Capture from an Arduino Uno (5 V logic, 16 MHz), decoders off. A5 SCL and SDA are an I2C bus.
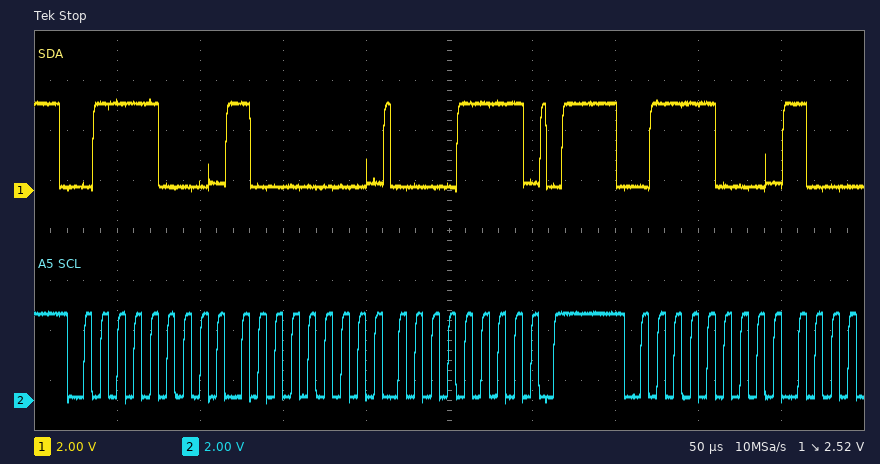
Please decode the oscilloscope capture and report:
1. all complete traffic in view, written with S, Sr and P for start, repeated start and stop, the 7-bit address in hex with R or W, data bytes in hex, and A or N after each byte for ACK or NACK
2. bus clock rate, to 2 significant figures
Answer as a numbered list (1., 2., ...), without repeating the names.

1. S 3CW A 80 A 0F A P S 3CW A
2. 100 kHz
